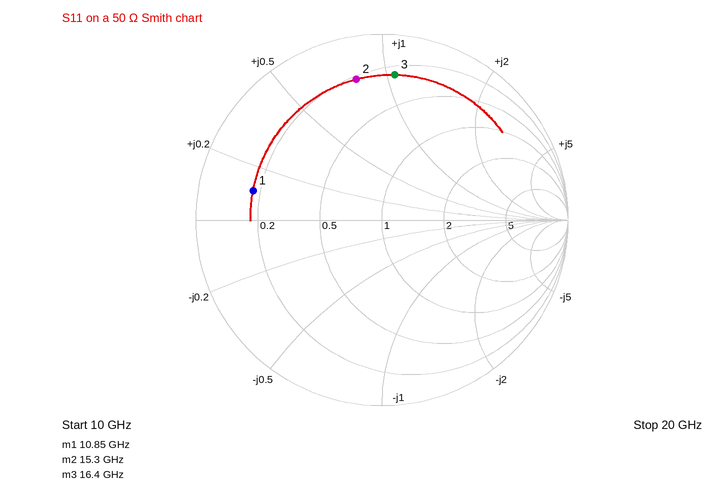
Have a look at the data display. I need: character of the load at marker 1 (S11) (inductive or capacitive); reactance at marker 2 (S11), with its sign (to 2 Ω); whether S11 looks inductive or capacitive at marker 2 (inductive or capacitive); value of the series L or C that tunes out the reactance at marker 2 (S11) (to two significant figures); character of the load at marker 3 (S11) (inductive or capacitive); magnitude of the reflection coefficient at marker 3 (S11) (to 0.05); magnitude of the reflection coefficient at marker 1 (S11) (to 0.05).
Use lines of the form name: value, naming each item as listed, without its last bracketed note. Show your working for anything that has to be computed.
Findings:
character of the load at marker 1 (S11): inductive
reactance at marker 2 (S11), with its sign: +40 Ω
whether S11 looks inductive or capacitive at marker 2: inductive
value of the series L or C that tunes out the reactance at marker 2 (S11): C = 1/(2π × 15.3 GHz × 40 Ω) ≈ 260 fF
character of the load at marker 3 (S11): inductive
magnitude of the reflection coefficient at marker 3 (S11): 0.80
magnitude of the reflection coefficient at marker 1 (S11): 0.70
